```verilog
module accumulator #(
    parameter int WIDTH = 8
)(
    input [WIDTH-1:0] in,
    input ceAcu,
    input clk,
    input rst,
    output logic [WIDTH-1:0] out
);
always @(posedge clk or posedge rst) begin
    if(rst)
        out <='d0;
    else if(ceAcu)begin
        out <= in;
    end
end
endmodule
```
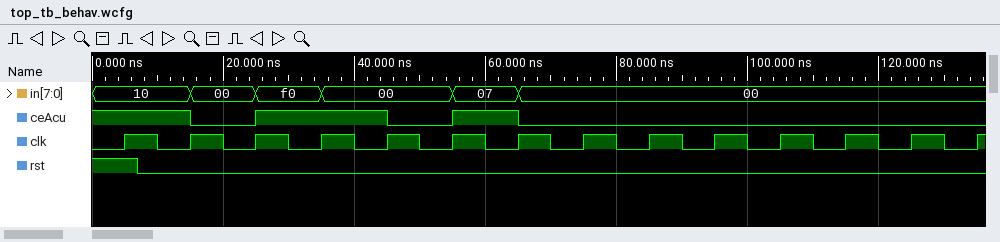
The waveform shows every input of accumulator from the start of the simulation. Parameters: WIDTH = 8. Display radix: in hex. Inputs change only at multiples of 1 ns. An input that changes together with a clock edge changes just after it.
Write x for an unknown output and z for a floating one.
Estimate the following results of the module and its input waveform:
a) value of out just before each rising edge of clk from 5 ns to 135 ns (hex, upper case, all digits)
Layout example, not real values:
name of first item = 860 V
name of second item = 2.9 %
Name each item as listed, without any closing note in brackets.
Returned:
value of out just before each rising edge of clk from 5 ns to 135 ns = 00, 00, 10, 10, F0, 00, 00, 07, 07, 07, 07, 07, 07, 07
